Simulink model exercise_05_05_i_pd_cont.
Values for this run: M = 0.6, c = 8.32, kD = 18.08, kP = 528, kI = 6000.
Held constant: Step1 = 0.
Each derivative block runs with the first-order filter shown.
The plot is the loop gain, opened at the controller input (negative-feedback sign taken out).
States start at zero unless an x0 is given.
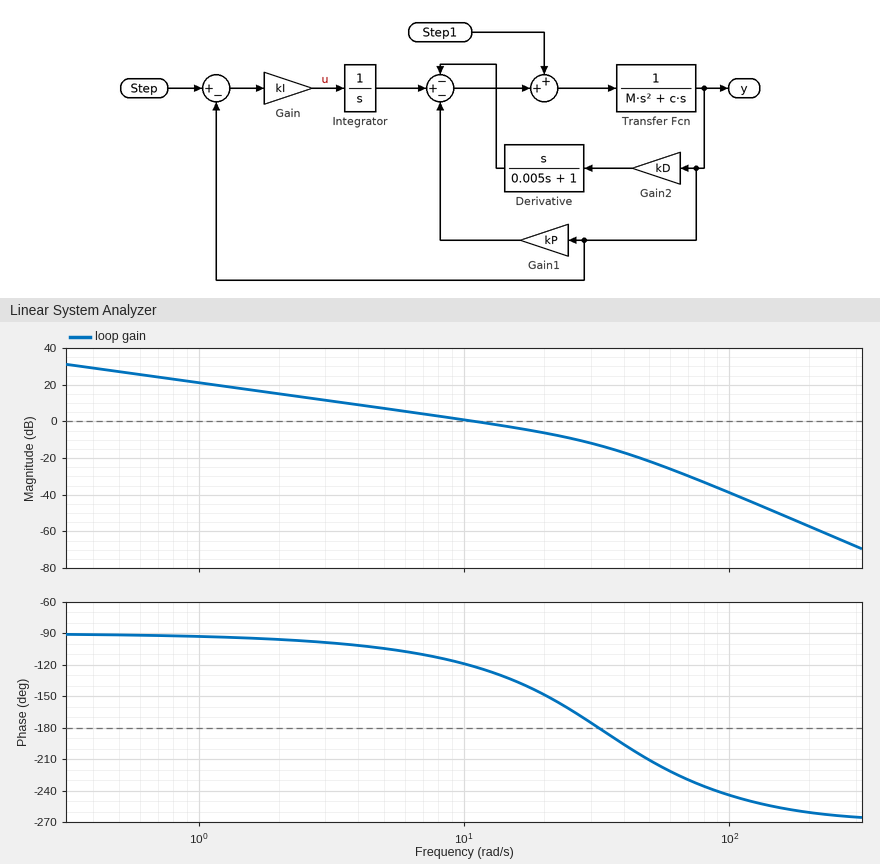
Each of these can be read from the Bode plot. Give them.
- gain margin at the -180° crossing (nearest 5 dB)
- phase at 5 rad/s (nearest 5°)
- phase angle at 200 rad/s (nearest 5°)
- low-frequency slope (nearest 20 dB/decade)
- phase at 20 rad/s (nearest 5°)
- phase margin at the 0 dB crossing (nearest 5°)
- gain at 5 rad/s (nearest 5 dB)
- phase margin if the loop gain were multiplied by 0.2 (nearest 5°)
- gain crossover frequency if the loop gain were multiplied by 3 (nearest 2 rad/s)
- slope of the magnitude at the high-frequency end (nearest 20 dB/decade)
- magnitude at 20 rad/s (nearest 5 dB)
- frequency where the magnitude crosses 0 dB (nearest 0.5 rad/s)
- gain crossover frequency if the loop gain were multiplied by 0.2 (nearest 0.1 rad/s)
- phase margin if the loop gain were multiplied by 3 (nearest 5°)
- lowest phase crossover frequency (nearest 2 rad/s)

15 dB
-105°
-260°
-20 dB/decade
-150°
60°
5 dB
85°
26 rad/s
-60 dB/decade
-5 dB
11.0 rad/s
2.3 rad/s
15°
32 rad/s
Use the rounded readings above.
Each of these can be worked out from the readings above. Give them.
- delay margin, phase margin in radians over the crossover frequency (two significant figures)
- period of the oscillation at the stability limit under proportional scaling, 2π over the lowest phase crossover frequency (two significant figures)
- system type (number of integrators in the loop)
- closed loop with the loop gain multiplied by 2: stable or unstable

0.095 s
0.20 s
1
stable
